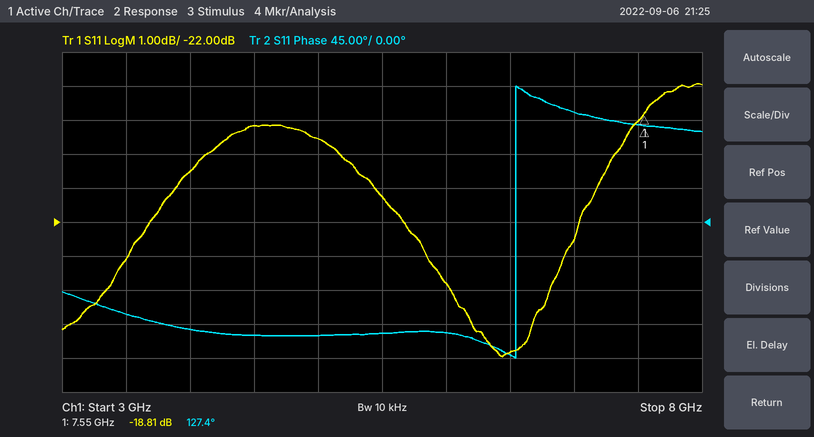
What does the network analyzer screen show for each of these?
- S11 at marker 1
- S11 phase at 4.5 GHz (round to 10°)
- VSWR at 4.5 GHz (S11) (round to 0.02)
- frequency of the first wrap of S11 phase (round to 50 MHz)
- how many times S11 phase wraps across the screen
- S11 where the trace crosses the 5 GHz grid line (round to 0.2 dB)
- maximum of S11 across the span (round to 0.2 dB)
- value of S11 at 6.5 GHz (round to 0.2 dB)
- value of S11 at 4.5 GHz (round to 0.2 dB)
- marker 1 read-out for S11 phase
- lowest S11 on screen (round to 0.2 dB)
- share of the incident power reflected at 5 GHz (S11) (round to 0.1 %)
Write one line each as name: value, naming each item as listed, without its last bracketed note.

S11 at marker 1: -18.81 dB
S11 phase at 4.5 GHz: -150°
VSWR at 4.5 GHz (S11): 1.24
frequency of the first wrap of S11 phase: 6.55 GHz
how many times S11 phase wraps across the screen: 1
S11 where the trace crosses the 5 GHz grid line: -19.6 dB
maximum of S11 across the span: -18.0 dB
value of S11 at 6.5 GHz: -25.8 dB
value of S11 at 4.5 GHz: -19.2 dB
marker 1 read-out for S11 phase: 127.4°
lowest S11 on screen: -26.0 dB
share of the incident power reflected at 5 GHz (S11): 1.1 %
